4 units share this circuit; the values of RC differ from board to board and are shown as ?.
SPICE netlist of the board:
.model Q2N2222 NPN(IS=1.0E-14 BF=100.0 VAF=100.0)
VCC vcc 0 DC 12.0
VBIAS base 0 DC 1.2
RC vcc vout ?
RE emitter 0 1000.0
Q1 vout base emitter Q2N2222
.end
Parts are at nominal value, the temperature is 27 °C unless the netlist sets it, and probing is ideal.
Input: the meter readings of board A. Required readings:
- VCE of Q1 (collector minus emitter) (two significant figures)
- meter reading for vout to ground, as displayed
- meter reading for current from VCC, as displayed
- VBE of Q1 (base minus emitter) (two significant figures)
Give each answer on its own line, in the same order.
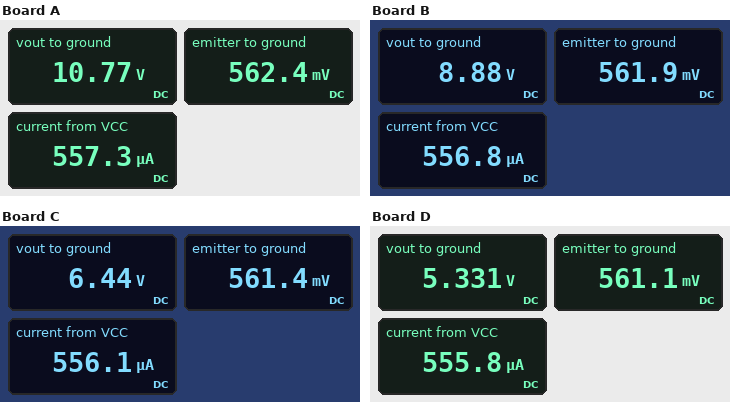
10 V
10.77 V
557.3 µA
640 mV
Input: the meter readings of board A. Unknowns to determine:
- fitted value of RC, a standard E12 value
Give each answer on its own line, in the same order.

2.2 kΩ
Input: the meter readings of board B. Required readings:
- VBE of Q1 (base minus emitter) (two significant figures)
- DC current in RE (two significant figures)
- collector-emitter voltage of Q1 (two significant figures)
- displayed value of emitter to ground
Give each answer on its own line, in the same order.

640 mV
560 µA
8.3 V
561.9 mV
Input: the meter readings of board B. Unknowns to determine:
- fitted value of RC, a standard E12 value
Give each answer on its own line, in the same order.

5.6 kΩ
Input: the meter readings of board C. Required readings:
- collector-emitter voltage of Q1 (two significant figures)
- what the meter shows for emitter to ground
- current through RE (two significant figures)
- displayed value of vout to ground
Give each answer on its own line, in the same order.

5.9 V
561.4 mV
560 µA
6.44 V
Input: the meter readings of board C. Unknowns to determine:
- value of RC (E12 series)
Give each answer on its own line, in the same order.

10 kΩ
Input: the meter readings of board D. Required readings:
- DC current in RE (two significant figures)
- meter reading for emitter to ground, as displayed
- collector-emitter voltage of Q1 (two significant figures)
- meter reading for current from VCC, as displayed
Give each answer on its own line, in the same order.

560 µA
561.1 mV
4.8 V
555.8 µA
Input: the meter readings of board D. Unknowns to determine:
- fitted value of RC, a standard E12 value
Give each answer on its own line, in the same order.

12 kΩ
